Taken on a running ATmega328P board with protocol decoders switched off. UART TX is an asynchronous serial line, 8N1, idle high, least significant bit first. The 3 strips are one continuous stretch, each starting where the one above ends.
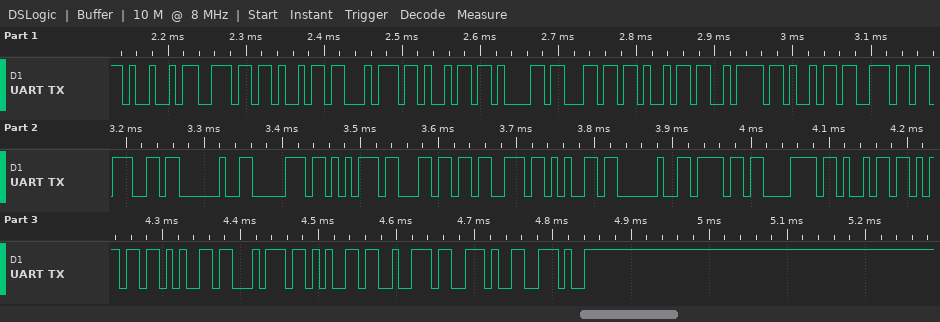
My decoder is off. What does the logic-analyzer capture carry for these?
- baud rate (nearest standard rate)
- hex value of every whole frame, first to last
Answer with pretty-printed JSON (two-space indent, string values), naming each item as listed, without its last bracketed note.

{
  "baud rate": "115200 baud",
  "hex value of every whole frame, first to last": "49 6E 69 74 69 61 6C 69 7A 69 6E 67 20 70 75 6C 73 65 20 6F 78 69 6D 65 74 65 72 2E 2E"
}
